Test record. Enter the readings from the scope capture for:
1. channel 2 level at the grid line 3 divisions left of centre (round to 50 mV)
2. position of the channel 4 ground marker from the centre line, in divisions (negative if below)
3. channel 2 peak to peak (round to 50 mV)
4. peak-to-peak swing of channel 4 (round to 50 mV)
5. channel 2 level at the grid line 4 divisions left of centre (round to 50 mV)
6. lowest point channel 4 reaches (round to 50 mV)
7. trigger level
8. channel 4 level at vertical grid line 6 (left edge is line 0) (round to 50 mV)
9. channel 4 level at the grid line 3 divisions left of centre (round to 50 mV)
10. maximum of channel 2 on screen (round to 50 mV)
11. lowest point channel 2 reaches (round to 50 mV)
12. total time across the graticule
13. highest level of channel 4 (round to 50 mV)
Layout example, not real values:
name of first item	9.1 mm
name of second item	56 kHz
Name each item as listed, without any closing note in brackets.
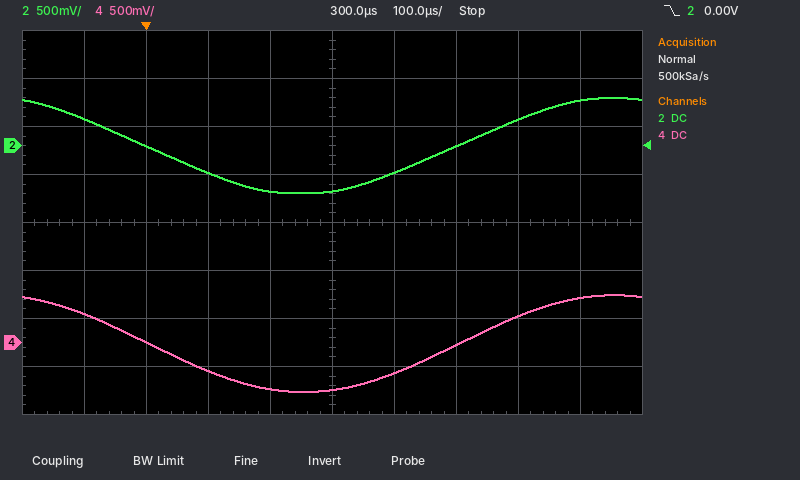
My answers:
channel 2 level at the grid line 3 divisions left of centre	0 mV
position of the channel 4 ground marker from the centre line, in divisions	-2.5 div
channel 2 peak to peak	1.00 V
peak-to-peak swing of channel 4	1.00 V
channel 2 level at the grid line 4 divisions left of centre	300 mV
lowest point channel 4 reaches	-500 mV
trigger level	0.00 V
channel 4 level at vertical grid line 6 (left edge is line 0)	-300 mV
channel 4 level at the grid line 3 divisions left of centre	0 mV
maximum of channel 2 on screen	500 mV
lowest point channel 2 reaches	-500 mV
total time across the graticule	1 ms
highest level of channel 4	500 mV
